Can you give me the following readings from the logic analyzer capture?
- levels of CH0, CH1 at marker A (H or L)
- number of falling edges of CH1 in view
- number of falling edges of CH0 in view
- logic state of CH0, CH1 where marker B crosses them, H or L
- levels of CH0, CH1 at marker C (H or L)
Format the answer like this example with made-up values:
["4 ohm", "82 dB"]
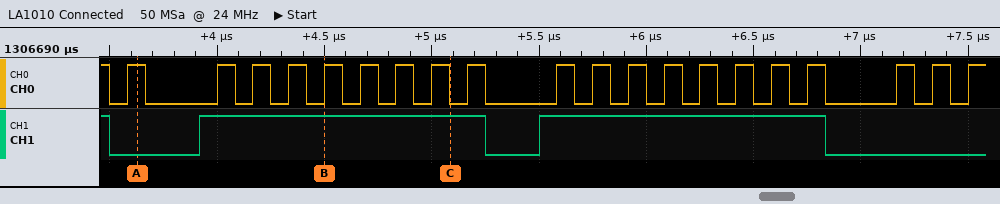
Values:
["CH0=H, CH1=L", "3", "20", "CH0=H, CH1=H", "CH0=L, CH1=H"]
